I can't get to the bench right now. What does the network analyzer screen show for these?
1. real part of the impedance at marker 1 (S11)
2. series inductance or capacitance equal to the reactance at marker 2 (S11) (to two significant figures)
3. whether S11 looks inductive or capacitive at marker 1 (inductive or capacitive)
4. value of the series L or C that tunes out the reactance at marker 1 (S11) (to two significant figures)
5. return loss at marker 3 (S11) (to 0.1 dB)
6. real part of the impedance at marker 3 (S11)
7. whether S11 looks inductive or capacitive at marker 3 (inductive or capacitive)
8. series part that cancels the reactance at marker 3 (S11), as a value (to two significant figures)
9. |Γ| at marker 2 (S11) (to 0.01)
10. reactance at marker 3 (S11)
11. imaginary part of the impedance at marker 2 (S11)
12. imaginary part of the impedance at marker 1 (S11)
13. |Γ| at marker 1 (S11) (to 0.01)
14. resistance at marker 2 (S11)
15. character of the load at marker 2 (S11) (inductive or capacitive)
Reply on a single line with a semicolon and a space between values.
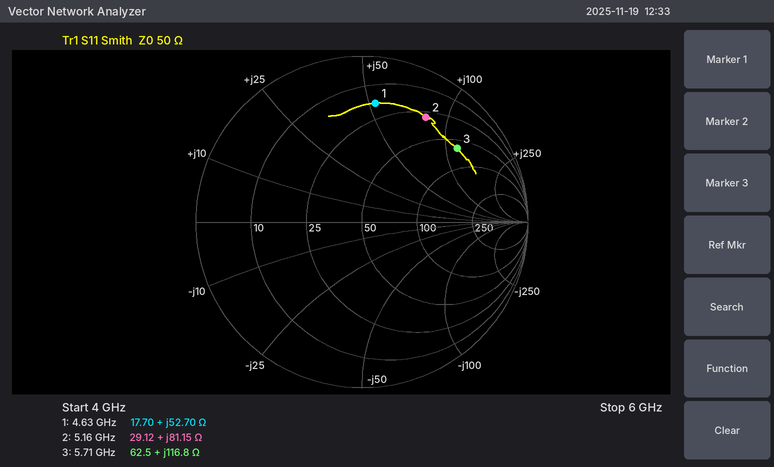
17.70 Ω; 2.5 nH; inductive; 650 fF; 2.8 dB; 62.5 Ω; inductive; 240 fF; 0.74; +116.8 Ω; +81.15 Ω; +52.70 Ω; 0.72; 29.12 Ω; inductive
